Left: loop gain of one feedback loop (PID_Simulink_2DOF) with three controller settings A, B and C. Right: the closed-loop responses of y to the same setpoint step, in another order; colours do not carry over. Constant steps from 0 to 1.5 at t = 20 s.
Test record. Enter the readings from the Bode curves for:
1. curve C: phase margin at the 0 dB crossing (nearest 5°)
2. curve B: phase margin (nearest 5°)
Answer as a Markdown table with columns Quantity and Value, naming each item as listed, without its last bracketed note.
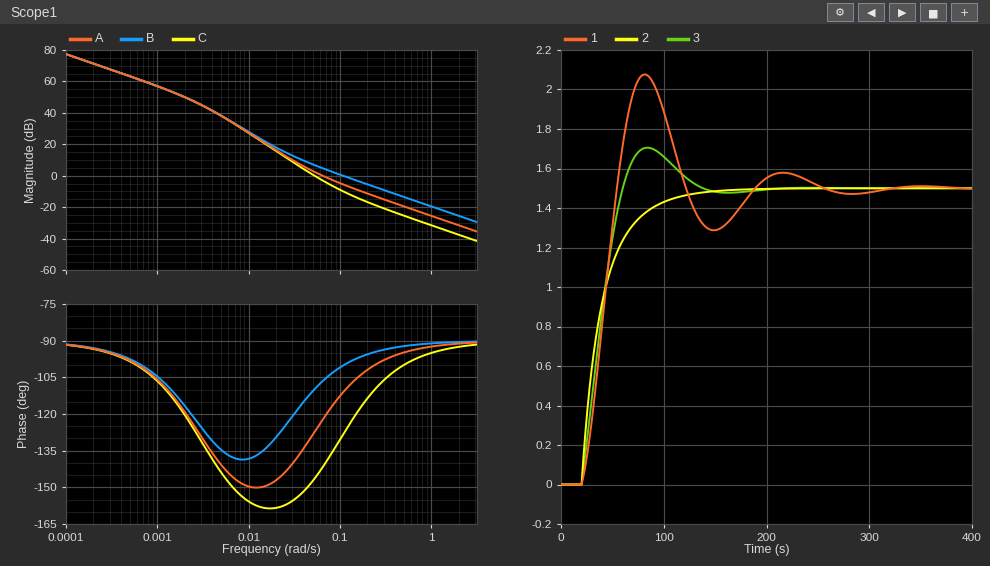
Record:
| Quantity | Value |
|---|---|
| curve C: phase margin at the 0 dB crossing | 35° |
| curve B: phase margin | 80° |
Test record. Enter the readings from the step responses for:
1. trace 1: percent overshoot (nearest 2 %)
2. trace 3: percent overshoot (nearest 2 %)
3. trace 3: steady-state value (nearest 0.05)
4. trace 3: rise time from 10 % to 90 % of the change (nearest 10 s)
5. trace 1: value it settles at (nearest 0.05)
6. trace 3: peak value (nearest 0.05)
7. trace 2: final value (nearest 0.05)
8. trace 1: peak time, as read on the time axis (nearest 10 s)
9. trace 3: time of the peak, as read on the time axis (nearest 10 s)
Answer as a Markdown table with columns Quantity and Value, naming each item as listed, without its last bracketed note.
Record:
| Quantity | Value |
|---|---|
| trace 1: percent overshoot | 38 % |
| trace 3: percent overshoot | 14 % |
| trace 3: steady-state value | 1.50 |
| trace 3: rise time from 10 % to 90 % of the change | 30 s |
| trace 1: value it settles at | 1.50 |
| trace 3: peak value | 1.70 |
| trace 2: final value | 1.50 |
| trace 1: peak time, as read on the time axis | 80 s |
| trace 3: time of the peak, as read on the time axis | 80 s |
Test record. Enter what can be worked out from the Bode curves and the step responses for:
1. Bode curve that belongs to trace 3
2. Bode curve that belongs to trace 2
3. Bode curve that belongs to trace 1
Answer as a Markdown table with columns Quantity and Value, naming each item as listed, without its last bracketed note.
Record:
| Quantity | Value |
|---|---|
| Bode curve that belongs to trace 3 | A |
| Bode curve that belongs to trace 2 | B |
| Bode curve that belongs to trace 1 | C |
